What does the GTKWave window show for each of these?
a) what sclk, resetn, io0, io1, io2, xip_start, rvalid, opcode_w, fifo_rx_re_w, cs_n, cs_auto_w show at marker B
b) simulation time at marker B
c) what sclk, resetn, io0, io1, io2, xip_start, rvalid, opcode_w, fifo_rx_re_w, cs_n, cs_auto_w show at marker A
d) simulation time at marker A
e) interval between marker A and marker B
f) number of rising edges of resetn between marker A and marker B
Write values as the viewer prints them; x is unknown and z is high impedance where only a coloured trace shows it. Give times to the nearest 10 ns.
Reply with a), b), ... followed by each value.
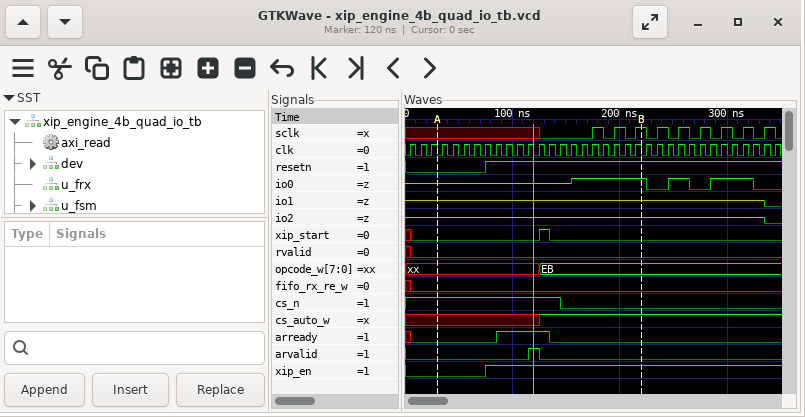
a) sclk=1, resetn=1, io0=1, io1=z, io2=z, xip_start=0, rvalid=0, opcode_w=EB, fifo_rx_re_w=0, cs_n=0, cs_auto_w=1
b) 220 ns
c) sclk=x, resetn=0, io0=z, io1=z, io2=z, xip_start=0, rvalid=0, opcode_w=xx, fifo_rx_re_w=0, cs_n=1, cs_auto_w=x
d) 30 ns
e) 190 ns
f) 1
